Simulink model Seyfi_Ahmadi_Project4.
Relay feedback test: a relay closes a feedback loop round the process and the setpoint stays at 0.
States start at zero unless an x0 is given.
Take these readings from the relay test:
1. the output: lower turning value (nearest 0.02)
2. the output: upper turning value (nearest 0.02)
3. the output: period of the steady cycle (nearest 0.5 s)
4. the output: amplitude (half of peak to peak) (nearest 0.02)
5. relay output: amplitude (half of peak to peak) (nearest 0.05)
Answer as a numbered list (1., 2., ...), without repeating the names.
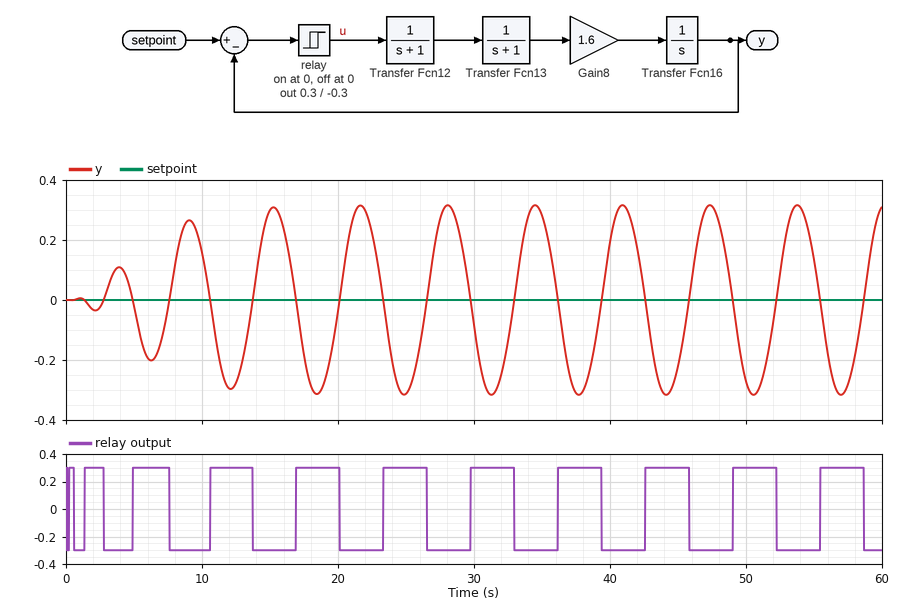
1. -0.32
2. 0.32
3. 6.5 s
4. 0.32
5. 0.30
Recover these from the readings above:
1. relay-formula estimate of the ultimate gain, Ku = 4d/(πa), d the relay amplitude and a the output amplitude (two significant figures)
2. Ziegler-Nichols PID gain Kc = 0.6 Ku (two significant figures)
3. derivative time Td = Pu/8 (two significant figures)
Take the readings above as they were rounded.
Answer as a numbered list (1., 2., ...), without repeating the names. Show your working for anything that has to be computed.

1. 4 × 0.3 / (π × 0.32) = 1.2
2. 0.6 × 1.2 = 0.72
3. 6.5 / 8 = 0.81 s
